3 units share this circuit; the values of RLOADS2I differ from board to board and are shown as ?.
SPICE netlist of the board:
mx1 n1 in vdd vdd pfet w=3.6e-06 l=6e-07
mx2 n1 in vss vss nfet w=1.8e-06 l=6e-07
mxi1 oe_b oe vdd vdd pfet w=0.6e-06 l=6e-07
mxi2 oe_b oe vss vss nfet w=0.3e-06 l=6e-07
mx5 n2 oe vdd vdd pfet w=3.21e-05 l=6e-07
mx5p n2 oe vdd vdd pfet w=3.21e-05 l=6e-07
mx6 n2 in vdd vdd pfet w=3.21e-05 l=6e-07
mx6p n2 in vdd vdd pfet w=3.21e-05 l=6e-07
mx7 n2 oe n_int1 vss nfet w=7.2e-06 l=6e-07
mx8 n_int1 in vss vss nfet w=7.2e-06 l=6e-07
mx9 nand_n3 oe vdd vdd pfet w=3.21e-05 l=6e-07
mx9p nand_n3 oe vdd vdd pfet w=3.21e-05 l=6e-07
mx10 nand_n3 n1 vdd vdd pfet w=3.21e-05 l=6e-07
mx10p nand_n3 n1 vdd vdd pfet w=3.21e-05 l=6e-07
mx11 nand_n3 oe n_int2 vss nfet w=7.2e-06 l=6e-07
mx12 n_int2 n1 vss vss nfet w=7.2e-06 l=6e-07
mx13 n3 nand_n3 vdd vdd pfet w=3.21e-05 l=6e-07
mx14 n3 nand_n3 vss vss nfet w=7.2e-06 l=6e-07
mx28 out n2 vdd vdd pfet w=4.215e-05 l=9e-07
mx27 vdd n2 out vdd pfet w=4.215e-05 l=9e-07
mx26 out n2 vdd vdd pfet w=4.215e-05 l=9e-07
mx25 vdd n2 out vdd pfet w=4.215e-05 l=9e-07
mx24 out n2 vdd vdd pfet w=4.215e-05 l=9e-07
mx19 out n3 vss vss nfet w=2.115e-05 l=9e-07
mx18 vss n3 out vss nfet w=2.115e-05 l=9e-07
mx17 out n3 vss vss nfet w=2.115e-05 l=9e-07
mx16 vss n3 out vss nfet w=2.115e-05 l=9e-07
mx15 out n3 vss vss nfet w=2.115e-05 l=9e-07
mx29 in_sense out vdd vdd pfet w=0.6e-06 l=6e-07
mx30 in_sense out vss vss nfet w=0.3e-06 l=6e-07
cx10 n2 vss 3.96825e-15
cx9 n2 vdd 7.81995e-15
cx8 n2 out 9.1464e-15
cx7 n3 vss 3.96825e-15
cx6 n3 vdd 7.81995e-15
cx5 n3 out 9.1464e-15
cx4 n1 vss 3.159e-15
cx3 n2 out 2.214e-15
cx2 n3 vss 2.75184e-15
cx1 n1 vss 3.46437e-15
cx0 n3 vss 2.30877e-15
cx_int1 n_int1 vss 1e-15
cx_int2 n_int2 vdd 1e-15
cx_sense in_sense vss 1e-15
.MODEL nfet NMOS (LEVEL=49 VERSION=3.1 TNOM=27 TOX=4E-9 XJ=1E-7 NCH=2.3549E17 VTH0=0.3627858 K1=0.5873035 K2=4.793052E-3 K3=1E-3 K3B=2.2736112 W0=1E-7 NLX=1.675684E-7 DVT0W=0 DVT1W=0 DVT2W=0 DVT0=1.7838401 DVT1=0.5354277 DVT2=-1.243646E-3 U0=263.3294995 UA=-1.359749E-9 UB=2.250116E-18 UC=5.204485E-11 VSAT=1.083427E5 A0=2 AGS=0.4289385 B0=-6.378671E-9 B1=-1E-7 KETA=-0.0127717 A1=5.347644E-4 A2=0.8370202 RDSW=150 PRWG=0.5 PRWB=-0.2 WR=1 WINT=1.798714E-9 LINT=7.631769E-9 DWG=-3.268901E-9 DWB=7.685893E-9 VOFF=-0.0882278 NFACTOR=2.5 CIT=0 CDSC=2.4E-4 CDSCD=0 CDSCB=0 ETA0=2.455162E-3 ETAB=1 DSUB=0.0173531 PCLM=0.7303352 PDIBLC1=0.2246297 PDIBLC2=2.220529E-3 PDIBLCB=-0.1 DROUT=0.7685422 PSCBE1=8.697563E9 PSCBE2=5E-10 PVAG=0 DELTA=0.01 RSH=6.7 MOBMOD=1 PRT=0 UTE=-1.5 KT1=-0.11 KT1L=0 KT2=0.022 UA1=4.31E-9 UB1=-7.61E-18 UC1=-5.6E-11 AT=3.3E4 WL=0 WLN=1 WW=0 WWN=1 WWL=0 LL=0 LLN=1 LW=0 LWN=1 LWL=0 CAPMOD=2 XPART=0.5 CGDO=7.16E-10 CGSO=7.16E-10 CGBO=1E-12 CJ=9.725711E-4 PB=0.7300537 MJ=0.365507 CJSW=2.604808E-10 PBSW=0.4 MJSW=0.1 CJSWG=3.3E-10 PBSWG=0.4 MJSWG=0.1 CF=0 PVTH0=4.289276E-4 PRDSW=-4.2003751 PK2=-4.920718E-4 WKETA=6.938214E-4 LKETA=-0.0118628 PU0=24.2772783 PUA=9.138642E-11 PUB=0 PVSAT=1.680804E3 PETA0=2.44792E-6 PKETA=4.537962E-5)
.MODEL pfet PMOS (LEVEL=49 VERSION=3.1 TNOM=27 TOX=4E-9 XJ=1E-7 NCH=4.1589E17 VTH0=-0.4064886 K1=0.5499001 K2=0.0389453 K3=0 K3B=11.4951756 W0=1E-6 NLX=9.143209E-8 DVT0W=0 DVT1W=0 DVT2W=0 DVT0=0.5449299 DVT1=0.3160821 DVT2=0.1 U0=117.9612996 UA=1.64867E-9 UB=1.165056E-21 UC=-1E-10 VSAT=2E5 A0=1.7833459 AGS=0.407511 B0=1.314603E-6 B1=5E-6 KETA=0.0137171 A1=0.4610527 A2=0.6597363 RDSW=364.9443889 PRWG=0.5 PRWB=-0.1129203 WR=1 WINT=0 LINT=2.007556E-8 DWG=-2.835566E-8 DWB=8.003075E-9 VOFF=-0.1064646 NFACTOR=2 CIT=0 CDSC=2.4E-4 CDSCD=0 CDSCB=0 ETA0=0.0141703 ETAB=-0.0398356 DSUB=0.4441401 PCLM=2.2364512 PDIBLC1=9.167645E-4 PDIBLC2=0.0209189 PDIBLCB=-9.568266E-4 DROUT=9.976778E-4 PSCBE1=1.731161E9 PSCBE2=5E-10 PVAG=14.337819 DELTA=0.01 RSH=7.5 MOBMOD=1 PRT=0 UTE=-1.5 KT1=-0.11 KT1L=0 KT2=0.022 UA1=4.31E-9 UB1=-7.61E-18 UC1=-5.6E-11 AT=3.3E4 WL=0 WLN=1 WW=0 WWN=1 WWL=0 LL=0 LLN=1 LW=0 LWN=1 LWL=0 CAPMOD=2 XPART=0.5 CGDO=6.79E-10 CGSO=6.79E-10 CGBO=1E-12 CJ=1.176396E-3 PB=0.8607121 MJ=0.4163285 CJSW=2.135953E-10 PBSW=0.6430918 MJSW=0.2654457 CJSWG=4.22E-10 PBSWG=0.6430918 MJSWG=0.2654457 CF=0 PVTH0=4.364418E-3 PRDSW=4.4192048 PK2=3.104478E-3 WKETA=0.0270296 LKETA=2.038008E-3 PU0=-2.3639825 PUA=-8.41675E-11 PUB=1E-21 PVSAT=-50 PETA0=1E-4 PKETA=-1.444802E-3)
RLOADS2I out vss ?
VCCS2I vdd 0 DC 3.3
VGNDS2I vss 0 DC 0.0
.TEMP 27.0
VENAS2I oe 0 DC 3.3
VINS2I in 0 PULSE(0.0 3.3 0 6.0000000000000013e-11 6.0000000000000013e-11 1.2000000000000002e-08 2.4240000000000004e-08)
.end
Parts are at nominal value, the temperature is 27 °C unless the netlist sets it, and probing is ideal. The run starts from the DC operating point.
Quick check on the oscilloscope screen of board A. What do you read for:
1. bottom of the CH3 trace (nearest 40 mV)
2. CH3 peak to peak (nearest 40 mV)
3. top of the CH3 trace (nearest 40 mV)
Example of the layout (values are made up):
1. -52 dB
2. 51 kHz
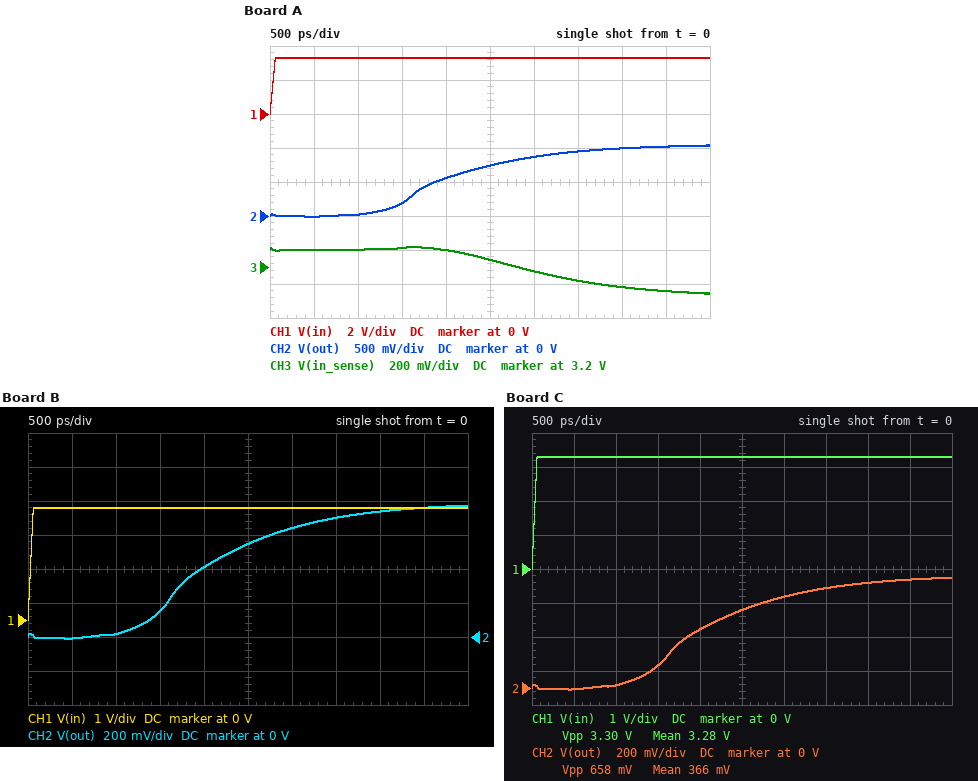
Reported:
1. 3.04 V
2. 280 mV
3. 3.32 V
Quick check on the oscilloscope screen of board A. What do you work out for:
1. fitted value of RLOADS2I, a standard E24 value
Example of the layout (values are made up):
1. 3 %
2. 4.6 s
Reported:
1. 33 Ω
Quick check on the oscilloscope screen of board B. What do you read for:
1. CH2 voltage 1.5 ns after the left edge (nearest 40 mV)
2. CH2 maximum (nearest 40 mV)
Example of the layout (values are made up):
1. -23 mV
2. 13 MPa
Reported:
1. 160 mV
2. 760 mV
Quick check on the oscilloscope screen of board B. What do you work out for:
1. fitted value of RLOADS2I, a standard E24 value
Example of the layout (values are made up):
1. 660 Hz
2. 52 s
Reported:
1. 24 Ω
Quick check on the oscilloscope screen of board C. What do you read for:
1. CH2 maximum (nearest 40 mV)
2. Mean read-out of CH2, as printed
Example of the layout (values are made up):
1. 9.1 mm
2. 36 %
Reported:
1. 640 mV
2. 366 mV
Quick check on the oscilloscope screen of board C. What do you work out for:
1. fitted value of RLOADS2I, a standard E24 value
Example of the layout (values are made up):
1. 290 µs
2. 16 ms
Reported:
1. 20 Ω
